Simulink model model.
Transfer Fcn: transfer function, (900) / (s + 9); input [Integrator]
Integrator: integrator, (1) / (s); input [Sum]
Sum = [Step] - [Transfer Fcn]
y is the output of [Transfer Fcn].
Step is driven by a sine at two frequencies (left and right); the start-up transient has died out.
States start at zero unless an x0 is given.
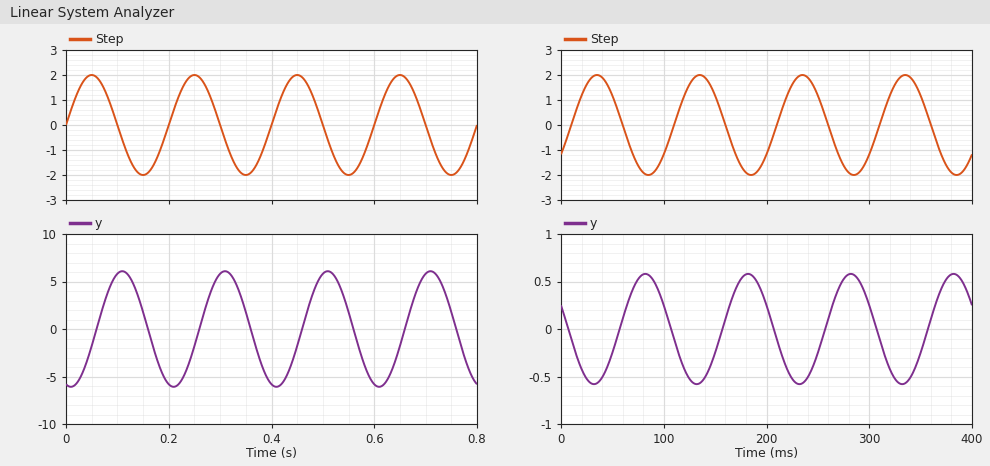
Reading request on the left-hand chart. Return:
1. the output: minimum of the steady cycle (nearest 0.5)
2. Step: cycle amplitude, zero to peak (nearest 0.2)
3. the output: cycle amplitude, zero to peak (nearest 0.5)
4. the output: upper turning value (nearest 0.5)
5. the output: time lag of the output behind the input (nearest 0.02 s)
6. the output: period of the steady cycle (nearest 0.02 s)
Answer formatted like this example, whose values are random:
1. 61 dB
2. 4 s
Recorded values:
1. -6.0
2. 2.0
3. 6.0
4. 6.0
5. 0.06 s
6. 0.20 s
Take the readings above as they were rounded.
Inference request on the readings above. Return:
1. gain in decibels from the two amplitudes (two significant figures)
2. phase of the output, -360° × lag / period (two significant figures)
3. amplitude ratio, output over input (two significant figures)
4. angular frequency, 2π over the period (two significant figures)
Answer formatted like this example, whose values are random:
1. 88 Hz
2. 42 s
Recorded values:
1. 9.5 dB
2. -110°
3. 3.0
4. 31 rad/s
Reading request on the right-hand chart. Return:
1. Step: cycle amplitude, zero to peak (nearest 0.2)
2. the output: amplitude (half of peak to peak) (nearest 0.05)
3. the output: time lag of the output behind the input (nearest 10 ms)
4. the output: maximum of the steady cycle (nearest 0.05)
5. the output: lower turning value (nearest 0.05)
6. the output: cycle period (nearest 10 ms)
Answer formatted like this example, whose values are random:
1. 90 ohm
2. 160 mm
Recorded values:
1. 2.0
2. 0.60
3. 50 ms
4. 0.60
5. -0.60
6. 100 ms
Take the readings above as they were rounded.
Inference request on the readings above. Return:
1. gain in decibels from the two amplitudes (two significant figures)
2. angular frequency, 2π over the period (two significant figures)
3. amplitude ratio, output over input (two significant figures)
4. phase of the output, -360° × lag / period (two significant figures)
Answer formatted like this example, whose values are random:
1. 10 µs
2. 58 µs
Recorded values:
1. -10 dB
2. 0.063 rad/ms
3. 0.30
4. -180°
